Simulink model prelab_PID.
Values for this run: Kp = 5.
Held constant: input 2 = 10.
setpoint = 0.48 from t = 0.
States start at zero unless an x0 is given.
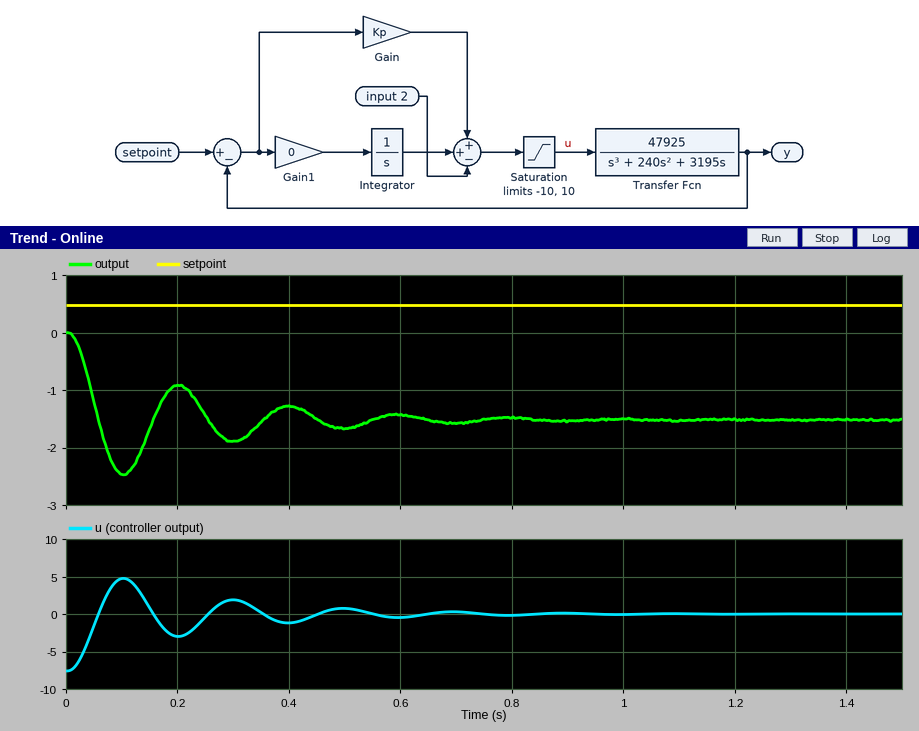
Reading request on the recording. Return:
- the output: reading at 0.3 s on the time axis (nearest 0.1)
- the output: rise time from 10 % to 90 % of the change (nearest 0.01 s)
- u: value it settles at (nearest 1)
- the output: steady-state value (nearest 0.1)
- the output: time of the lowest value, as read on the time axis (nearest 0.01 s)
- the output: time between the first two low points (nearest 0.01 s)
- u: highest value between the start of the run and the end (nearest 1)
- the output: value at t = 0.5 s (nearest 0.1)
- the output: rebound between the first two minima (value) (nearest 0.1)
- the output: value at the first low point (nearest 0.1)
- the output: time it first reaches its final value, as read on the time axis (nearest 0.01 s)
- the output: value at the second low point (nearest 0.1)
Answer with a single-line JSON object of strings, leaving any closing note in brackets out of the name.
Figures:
{"the output: reading at 0.3 s on the time axis": "-1.9", "the output: rise time from 10 % to 90 % of the change": "0.04 s", "u: value it settles at": "0", "the output: steady-state value": "-1.5", "the output: time of the lowest value, as read on the time axis": "0.10 s", "the output: time between the first two low points": "0.20 s", "u: highest value between the start of the run and the end": "5", "the output: value at t = 0.5 s": "-1.7", "the output: rebound between the first two minima (value)": "-0.9", "the output: value at the first low point": "-2.5", "the output: time it first reaches its final value, as read on the time axis": "0.06 s", "the output: value at the second low point": "-1.9"}
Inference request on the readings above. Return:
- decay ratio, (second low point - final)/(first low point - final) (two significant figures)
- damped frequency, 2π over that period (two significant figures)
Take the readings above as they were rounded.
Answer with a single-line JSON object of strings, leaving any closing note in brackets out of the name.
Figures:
{"decay ratio, (second low point - final)/(first low point - final)": "0.40", "damped frequency, 2π over that period": "31 rad/s"}
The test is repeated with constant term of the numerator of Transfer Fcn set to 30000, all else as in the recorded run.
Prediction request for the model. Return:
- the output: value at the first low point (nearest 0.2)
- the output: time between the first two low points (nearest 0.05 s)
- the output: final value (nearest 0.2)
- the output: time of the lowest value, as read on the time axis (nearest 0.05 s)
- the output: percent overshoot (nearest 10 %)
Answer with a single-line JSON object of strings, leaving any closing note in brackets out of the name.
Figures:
{"the output: value at the first low point": "-2.2", "the output: time between the first two low points": "0.25 s", "the output: final value": "-1.6", "the output: time of the lowest value, as read on the time axis": "0.15 s", "the output: percent overshoot": "50 %"}
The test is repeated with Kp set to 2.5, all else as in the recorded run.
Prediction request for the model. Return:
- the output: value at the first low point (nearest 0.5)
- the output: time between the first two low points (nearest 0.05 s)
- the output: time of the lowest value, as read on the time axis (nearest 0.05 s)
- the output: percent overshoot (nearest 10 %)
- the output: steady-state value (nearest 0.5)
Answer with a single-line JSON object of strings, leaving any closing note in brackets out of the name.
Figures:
{"the output: value at the first low point": "-5.0", "the output: time between the first two low points": "0.30 s", "the output: time of the lowest value, as read on the time axis": "0.15 s", "the output: percent overshoot": "40 %", "the output: steady-state value": "-3.5"}
